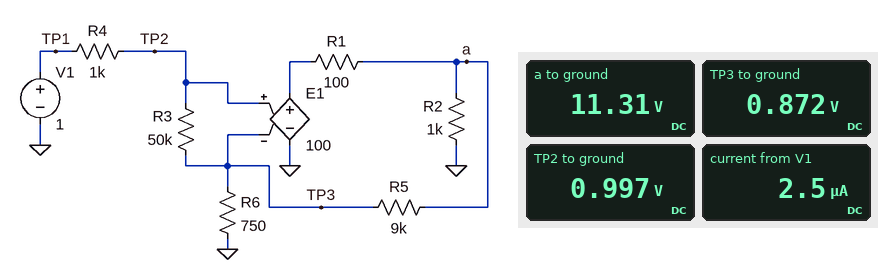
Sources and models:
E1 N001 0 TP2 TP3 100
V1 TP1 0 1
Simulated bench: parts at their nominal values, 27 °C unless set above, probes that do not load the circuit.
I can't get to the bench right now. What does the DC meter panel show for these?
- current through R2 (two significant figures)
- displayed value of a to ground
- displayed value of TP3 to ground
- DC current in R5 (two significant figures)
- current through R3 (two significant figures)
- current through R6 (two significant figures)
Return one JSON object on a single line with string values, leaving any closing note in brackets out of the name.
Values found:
{"current through R2": "11 mA", "displayed value of a to ground": "11.31 V", "displayed value of TP3 to ground": "0.872 V", "DC current in R5": "1.2 mA", "current through R3": "2.5 µA", "current through R6": "1.2 mA"}
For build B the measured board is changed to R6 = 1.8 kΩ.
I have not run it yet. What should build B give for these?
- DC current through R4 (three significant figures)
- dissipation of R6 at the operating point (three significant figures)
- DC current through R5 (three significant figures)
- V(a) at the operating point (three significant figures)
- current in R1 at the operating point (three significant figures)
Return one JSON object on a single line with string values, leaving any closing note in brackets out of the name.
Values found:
{"DC current through R4": "1.24 µA", "dissipation of R6 at the operating point": "487 µW", "DC current through R5": "519 µA", "V(a) at the operating point": "5.61 V", "current in R1 at the operating point": "6.13 mA"}
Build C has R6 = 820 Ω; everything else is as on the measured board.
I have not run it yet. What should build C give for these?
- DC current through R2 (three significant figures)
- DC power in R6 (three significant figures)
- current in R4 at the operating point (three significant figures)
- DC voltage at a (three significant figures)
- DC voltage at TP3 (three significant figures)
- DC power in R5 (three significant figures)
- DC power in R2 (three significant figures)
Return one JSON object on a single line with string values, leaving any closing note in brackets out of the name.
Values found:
{"DC current through R2": "10.5 mA", "DC power in R6": "946 µW", "current in R4 at the operating point": "2.34 µA", "DC voltage at a": "10.5 V", "DC voltage at TP3": "881 mV", "DC power in R5": "10.3 mW", "DC power in R2": "111 mW"}
